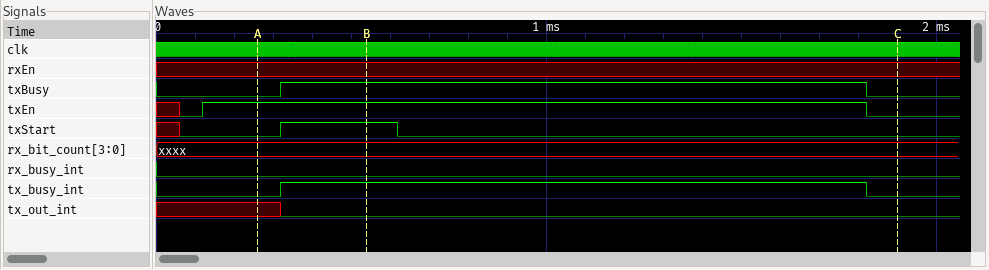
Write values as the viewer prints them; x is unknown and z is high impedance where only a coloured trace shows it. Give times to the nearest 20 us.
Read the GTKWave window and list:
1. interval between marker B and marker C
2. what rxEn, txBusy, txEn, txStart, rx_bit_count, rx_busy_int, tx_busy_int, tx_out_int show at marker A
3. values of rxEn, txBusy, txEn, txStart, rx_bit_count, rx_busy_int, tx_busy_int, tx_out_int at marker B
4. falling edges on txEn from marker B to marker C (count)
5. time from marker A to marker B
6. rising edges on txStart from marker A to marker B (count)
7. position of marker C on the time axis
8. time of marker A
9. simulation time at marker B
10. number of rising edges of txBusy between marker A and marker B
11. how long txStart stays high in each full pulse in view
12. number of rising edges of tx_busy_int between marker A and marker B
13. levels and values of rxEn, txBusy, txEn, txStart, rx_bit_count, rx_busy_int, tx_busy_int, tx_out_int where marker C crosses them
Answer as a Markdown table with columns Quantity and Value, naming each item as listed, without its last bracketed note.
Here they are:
| Quantity | Value |
|---|---|
| interval between marker B and marker C | 1360 us |
| what rxEn, txBusy, txEn, txStart, rx_bit_count, rx_busy_int, tx_busy_int, tx_out_int show at marker A | rxEn=x, txBusy=0, txEn=1, txStart=0, rx_bit_count=xxxx, rx_busy_int=0, tx_busy_int=0, tx_out_int=x |
| values of rxEn, txBusy, txEn, txStart, rx_bit_count, rx_busy_int, tx_busy_int, tx_out_int at marker B | rxEn=x, txBusy=1, txEn=1, txStart=1, rx_bit_count=xxxx, rx_busy_int=0, tx_busy_int=1, tx_out_int=0 |
| falling edges on txEn from marker B to marker C | 1 |
| time from marker A to marker B | 280 us |
| rising edges on txStart from marker A to marker B | 1 |
| position of marker C on the time axis | 1900 us |
| time of marker A | 260 us |
| simulation time at marker B | 540 us |
| number of rising edges of txBusy between marker A and marker B | 1 |
| how long txStart stays high in each full pulse in view | 300 us |
| number of rising edges of tx_busy_int between marker A and marker B | 1 |
| levels and values of rxEn, txBusy, txEn, txStart, rx_bit_count, rx_busy_int, tx_busy_int, tx_out_int where marker C crosses them | rxEn=x, txBusy=0, txEn=0, txStart=0, rx_bit_count=xxxx, rx_busy_int=0, tx_busy_int=0, tx_out_int=0 |
